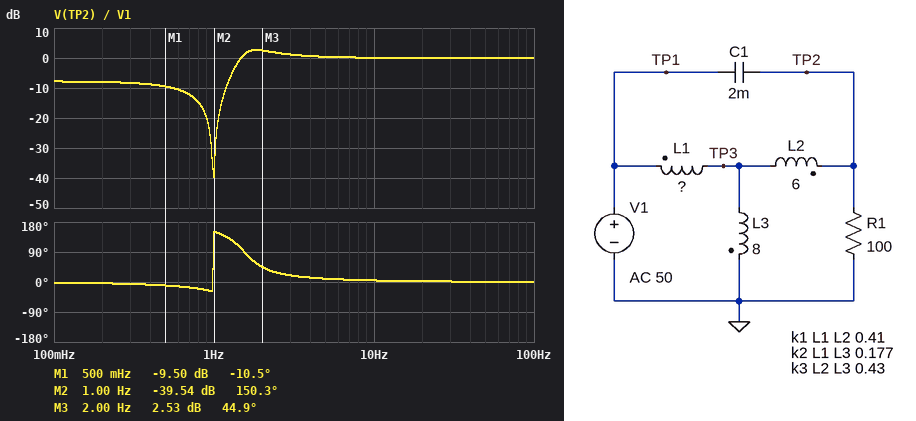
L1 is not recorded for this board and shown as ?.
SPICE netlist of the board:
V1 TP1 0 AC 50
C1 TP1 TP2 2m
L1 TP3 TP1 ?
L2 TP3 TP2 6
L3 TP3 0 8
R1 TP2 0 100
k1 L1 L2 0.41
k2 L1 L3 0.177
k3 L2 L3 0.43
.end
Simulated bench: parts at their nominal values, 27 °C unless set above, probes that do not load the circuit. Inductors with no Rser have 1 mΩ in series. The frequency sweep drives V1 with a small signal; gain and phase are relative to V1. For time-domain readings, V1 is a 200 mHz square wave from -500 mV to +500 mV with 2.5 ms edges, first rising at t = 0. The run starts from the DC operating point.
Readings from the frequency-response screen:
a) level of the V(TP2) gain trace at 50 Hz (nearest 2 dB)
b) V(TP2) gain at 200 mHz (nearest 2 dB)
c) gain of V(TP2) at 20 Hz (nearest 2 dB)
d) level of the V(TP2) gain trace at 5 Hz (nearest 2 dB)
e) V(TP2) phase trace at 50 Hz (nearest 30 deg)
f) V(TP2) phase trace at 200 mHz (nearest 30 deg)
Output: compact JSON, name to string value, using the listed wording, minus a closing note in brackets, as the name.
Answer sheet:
{"level of the V(TP2) gain trace at 50 Hz": "0 dB", "V(TP2) gain at 200 mHz": "-8 dB", "gain of V(TP2) at 20 Hz": "0 dB", "level of the V(TP2) gain trace at 5 Hz": "0 dB", "V(TP2) phase trace at 50 Hz": "0 deg", "V(TP2) phase trace at 200 mHz": "0 deg"}
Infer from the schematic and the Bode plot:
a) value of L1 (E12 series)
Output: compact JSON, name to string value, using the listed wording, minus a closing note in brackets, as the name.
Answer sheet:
{"value of L1": "12 H"}
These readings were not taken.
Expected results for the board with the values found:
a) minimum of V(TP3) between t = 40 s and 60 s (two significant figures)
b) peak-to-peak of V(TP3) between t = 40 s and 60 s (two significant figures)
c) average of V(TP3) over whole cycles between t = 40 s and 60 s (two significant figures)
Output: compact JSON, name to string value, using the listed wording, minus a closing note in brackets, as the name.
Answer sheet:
{"minimum of V(TP3) between t = 40 s and 60 s": "-520 mV", "peak-to-peak of V(TP3) between t = 40 s and 60 s": "920 mV", "average of V(TP3) over whole cycles between t = 40 s and 60 s": "-60 mV"}
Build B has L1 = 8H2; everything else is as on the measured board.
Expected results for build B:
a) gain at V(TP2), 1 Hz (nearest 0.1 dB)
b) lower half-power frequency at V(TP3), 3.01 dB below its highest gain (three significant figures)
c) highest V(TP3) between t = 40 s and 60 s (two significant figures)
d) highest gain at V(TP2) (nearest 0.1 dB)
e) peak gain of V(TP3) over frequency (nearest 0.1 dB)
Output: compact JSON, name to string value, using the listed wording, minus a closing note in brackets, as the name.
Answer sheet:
{"gain at V(TP2), 1 Hz": "-17.0 dB", "lower half-power frequency at V(TP3), 3.01 dB below its highest gain": "1.63 Hz", "highest V(TP3) between t = 40 s and 60 s": "430 mV", "highest gain at V(TP2)": "2.2 dB", "peak gain of V(TP3) over frequency": "-2.6 dB"}
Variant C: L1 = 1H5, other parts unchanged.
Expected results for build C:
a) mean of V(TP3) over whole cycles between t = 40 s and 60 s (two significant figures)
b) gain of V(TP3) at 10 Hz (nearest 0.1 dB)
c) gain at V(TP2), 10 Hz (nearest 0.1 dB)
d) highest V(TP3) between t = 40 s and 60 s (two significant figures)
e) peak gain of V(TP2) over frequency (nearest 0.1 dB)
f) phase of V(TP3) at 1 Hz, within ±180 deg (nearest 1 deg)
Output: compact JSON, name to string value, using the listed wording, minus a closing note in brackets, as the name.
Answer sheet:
{"mean of V(TP3) over whole cycles between t = 40 s and 60 s": "190 mV", "gain of V(TP3) at 10 Hz": "-1.0 dB", "gain at V(TP2), 10 Hz": "0.1 dB", "highest V(TP3) between t = 40 s and 60 s": "640 mV", "peak gain of V(TP2) over frequency": "0.9 dB", "phase of V(TP3) at 1 Hz, within ±180 deg": "0 deg"}
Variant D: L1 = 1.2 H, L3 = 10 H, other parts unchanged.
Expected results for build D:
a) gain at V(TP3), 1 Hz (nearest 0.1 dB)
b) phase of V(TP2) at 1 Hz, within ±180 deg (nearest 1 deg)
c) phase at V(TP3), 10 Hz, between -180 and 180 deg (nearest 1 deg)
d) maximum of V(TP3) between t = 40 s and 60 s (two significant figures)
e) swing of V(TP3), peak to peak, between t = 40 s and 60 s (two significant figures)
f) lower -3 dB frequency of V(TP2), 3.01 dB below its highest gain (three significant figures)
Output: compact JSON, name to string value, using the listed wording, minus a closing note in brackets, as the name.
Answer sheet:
{"gain at V(TP3), 1 Hz": "-0.5 dB", "phase of V(TP2) at 1 Hz, within ±180 deg": "-22 deg", "phase at V(TP3), 10 Hz, between -180 and 180 deg": "0 deg", "maximum of V(TP3) between t = 40 s and 60 s": "690 mV", "swing of V(TP3), peak to peak, between t = 40 s and 60 s": "950 mV", "lower -3 dB frequency of V(TP2), 3.01 dB below its highest gain": "1.81 Hz"}
